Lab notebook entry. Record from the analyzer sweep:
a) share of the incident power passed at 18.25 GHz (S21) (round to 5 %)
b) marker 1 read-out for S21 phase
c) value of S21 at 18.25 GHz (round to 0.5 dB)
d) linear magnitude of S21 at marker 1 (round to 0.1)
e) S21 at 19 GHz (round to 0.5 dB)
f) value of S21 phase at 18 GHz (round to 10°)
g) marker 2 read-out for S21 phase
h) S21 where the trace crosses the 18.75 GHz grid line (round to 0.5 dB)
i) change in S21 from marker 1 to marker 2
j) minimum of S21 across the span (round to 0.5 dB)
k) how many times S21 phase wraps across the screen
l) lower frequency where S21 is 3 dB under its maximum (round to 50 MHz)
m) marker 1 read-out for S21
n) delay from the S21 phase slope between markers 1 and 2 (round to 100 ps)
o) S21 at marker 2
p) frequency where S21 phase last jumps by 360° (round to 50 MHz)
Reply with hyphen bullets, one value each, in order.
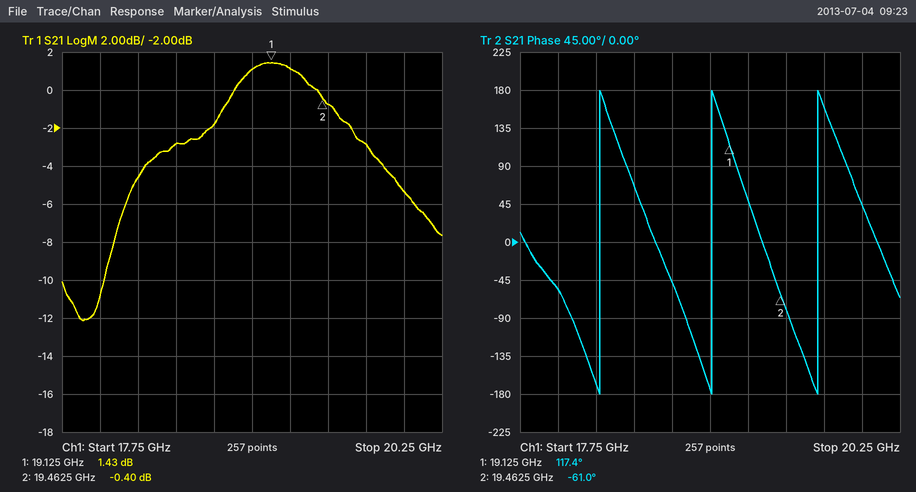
- 35 %
- 117.4°
- -4.5 dB
- 1.2
- 1.0 dB
- -60°
- -61.0°
- -2.0 dB
- -1.83 dB
- -12.0 dB
- 3
- 18.75 GHz
- 1.43 dB
- 1.5 ns
- -0.40 dB
- 19.70 GHz
